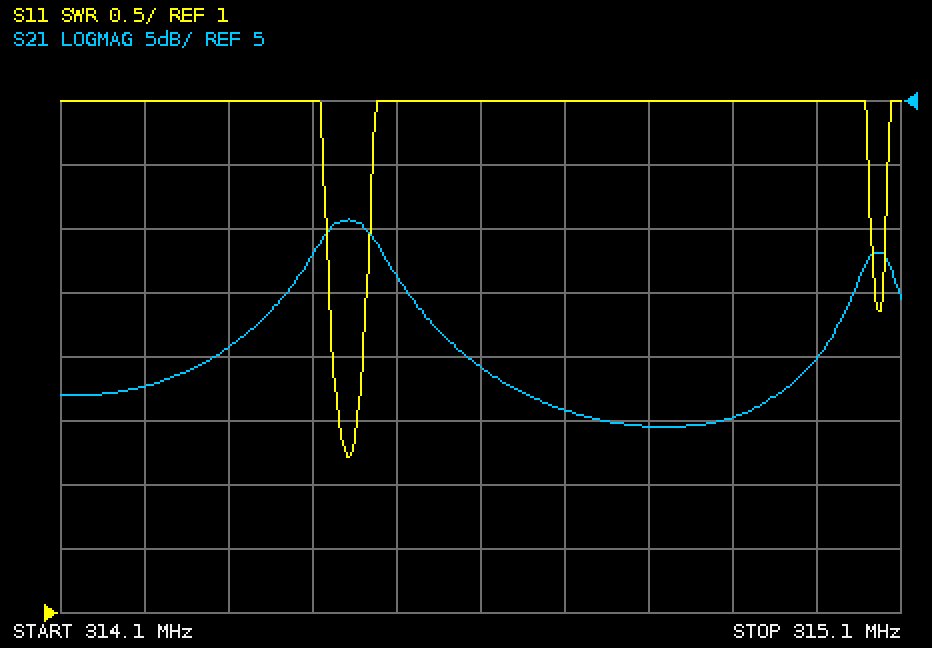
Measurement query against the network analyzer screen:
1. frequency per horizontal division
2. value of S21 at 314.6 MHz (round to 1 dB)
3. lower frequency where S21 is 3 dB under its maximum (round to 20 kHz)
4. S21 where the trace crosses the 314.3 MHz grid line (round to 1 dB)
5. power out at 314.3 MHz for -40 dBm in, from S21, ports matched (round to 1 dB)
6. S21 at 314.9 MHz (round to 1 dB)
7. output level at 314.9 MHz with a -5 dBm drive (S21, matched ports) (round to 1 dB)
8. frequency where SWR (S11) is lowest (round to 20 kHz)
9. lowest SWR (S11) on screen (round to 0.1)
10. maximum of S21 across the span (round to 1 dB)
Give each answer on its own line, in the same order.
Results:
100 kHz
-16 dB
314.40 MHz
-14 dB
-54 dBm
-20 dB
-25 dBm
314.44 MHz
2.2
-4 dB
